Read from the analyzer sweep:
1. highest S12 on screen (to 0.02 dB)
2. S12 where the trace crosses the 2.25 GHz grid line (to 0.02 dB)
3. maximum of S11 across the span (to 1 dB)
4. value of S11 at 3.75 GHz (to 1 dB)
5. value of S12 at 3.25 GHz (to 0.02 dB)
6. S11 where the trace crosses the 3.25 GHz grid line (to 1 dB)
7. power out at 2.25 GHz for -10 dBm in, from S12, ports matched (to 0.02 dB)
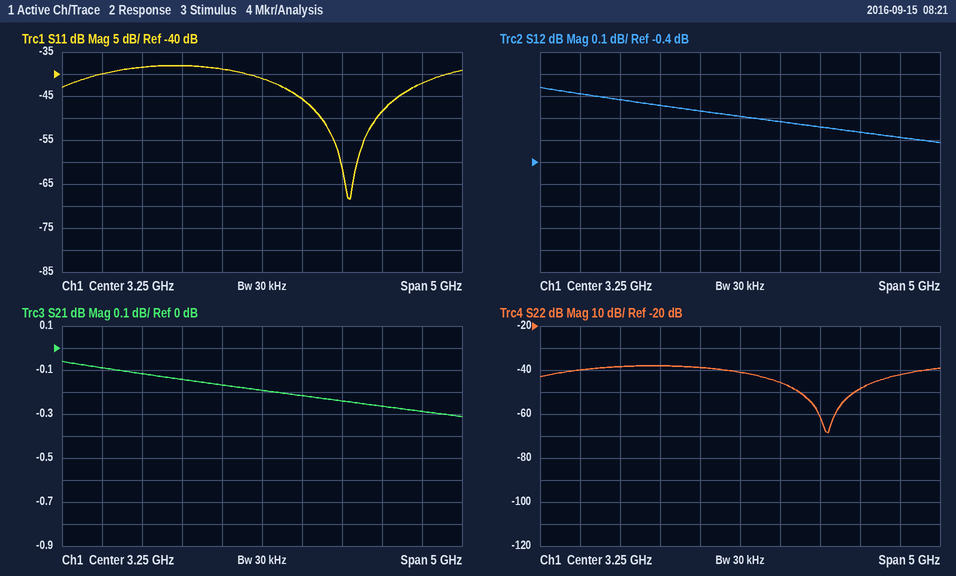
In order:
-0.06 dB
-0.14 dB
-38 dB
-46 dB
-0.20 dB
-41 dB
-10.14 dBm
